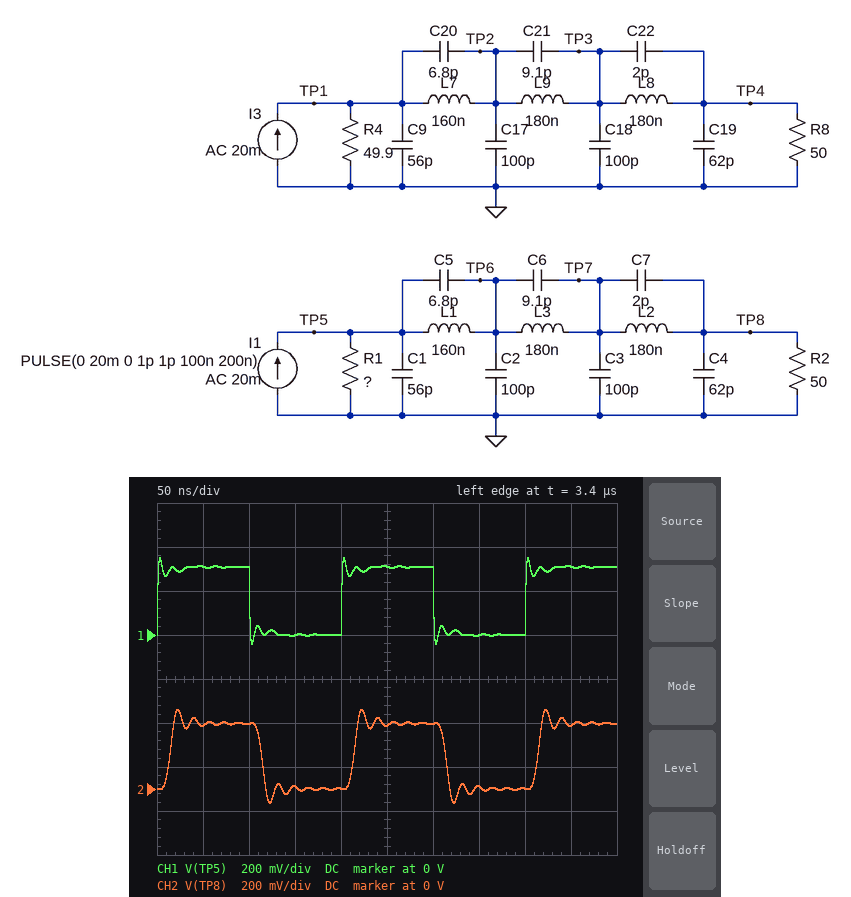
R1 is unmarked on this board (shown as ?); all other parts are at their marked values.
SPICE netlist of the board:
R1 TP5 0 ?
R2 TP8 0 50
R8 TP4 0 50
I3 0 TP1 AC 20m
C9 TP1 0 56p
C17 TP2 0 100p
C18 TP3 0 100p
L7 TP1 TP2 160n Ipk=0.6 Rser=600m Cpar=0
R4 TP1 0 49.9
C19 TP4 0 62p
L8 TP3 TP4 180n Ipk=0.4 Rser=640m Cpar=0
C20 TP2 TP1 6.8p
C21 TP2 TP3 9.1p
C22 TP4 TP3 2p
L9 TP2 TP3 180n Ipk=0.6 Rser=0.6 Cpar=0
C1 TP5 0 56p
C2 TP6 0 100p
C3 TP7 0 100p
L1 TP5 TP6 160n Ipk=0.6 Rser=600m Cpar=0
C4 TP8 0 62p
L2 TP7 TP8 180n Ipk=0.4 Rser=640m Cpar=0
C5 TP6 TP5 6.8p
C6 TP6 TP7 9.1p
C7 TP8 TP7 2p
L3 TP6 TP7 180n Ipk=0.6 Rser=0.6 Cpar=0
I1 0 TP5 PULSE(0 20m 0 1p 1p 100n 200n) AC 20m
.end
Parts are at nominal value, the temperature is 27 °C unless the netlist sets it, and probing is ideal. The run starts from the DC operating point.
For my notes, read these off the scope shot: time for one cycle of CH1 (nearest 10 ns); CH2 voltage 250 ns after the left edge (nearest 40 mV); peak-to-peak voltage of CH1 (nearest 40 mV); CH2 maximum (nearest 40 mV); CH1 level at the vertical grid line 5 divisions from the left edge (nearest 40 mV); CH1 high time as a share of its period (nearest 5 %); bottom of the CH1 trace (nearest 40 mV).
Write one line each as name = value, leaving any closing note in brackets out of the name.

time for one cycle of CH1 = 200 ns
CH2 voltage 250 ns after the left edge = 280 mV
peak-to-peak voltage of CH1 = 400 mV
CH2 maximum = 360 mV
CH1 level at the vertical grid line 5 divisions from the left edge = 320 mV
CH1 high time as a share of its period = 50 %
bottom of the CH1 trace = -40 mV
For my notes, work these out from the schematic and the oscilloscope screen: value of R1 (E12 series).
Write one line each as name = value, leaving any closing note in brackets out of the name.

value of R1 = 22 Ω
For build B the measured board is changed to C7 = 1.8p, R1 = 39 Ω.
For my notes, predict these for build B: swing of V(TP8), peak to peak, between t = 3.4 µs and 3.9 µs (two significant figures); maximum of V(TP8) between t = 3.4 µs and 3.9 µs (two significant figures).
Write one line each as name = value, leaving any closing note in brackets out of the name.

swing of V(TP8), peak to peak, between t = 3.4 µs and 3.9 µs = 590 mV
maximum of V(TP8) between t = 3.4 µs and 3.9 µs = 510 mV
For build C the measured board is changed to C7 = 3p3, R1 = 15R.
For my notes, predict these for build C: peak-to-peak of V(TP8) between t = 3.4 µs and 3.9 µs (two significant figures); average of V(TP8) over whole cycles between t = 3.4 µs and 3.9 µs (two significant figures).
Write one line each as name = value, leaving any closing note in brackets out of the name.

peak-to-peak of V(TP8) between t = 3.4 µs and 3.9 µs = 330 mV
average of V(TP8) over whole cycles between t = 3.4 µs and 3.9 µs = 110 mV
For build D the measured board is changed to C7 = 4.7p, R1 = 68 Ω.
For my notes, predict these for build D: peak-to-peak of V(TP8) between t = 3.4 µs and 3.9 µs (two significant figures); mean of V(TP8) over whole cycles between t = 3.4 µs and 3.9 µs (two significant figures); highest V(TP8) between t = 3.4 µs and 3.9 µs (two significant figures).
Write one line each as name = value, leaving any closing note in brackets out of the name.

peak-to-peak of V(TP8) between t = 3.4 µs and 3.9 µs = 760 mV
mean of V(TP8) over whole cycles between t = 3.4 µs and 3.9 µs = 280 mV
highest V(TP8) between t = 3.4 µs and 3.9 µs = 660 mV
